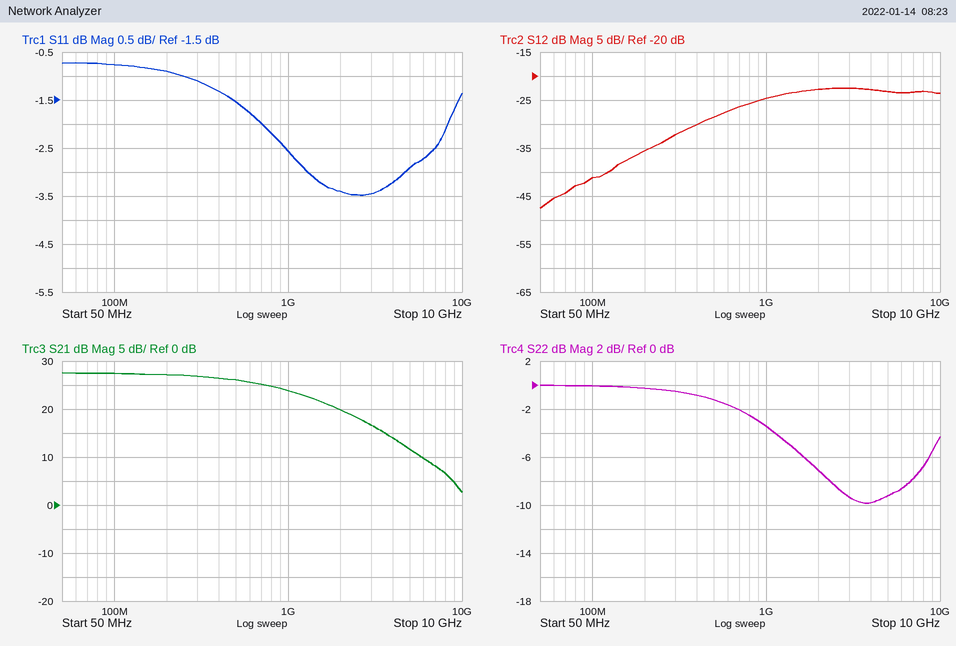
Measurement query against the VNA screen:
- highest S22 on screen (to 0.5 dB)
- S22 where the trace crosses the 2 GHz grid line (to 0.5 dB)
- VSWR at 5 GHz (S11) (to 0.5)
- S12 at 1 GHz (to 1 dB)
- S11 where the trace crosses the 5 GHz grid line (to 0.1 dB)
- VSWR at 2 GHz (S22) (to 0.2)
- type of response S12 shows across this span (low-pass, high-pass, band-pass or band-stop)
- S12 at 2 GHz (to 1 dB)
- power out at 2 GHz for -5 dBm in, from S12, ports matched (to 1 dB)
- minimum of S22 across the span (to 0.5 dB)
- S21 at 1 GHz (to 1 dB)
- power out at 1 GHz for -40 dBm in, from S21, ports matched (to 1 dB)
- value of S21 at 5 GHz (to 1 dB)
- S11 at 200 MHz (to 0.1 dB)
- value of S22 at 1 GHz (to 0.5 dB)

0.0 dB
-7.0 dB
6.0
-25 dB
-2.9 dB
2.6
high-pass
-23 dB
-28 dBm
-10.0 dB
24 dB
-16 dBm
12 dB
-0.9 dB
-3.5 dB
